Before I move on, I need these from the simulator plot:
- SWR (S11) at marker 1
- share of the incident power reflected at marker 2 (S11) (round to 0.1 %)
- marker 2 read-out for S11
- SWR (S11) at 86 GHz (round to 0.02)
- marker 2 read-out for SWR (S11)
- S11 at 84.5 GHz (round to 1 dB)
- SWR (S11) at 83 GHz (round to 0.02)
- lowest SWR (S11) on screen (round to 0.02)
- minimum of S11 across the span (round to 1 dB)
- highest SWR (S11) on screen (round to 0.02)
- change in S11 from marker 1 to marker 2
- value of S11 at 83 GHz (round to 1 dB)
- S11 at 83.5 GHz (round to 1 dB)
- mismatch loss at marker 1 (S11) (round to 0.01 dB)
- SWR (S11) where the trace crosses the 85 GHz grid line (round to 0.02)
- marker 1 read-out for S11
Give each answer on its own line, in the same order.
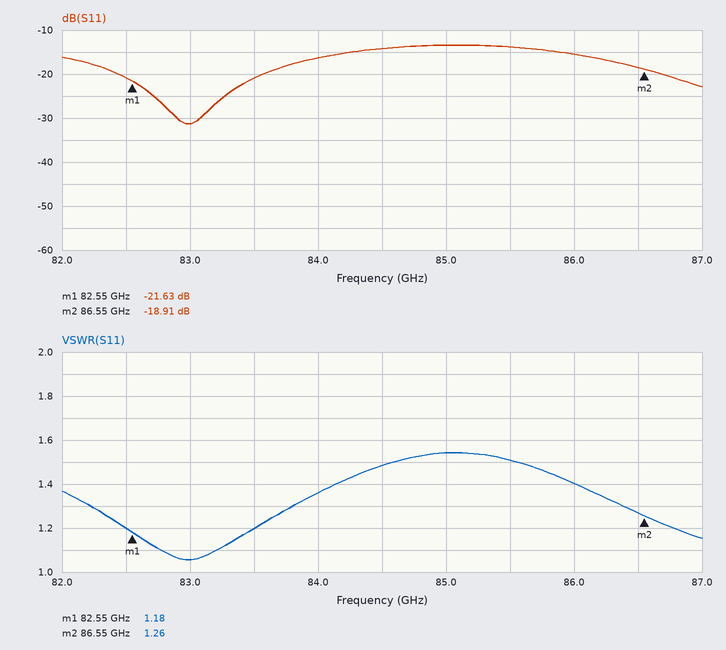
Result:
1.18
1.3 %
-18.91 dB
1.40
1.26
-14 dB
1.06
1.06
-31 dB
1.54
2.72 dB
-31 dB
-21 dB
0.03 dB
1.54
-21.63 dB
